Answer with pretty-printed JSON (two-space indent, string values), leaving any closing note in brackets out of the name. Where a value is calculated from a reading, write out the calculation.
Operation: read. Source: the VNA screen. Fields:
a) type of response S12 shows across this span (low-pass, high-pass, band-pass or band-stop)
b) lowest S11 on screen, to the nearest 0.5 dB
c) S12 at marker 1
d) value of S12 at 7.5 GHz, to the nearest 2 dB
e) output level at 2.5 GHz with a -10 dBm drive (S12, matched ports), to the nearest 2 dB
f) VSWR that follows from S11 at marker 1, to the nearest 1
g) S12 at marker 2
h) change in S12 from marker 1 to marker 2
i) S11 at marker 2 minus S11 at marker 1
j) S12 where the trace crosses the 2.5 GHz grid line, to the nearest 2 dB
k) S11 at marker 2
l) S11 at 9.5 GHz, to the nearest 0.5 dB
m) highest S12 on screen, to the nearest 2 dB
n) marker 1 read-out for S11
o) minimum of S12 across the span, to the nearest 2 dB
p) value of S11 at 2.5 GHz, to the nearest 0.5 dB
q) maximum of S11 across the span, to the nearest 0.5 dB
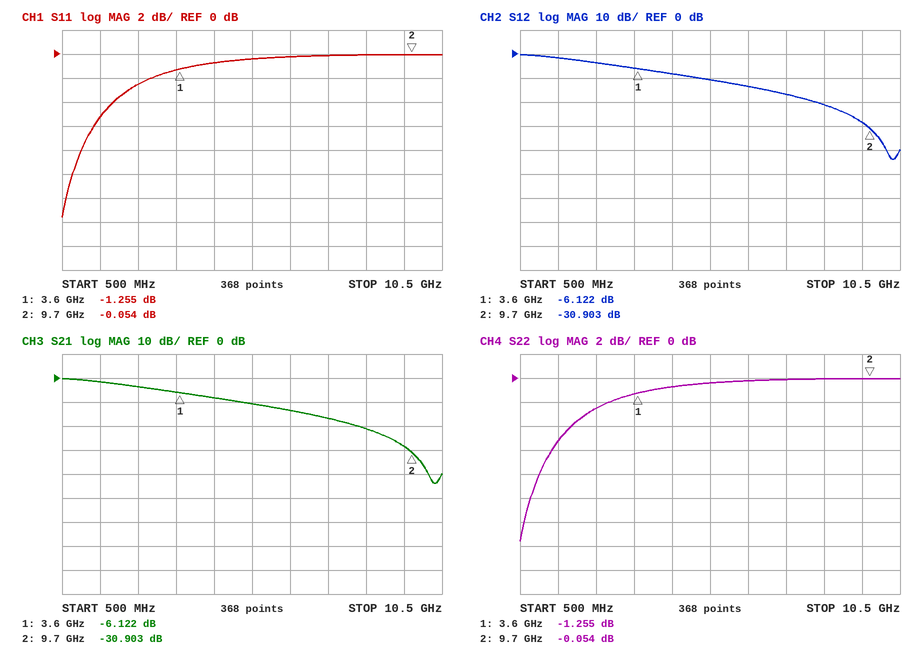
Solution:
{
  "type of response S12 shows across this span": "low-pass",
  "lowest S11 on screen, to the nearest 0.5 dB": "-13.5 dB",
  "S12 at marker 1": "-6.122 dB",
  "value of S12 at 7.5 GHz, to the nearest 2 dB": "-16 dB",
  "output level at 2.5 GHz with a -10 dBm drive (S12, matched ports), to the nearest 2 dB": "-10 dBm + (-4 dB) = -14 dBm",
  "VSWR that follows from S11 at marker 1, to the nearest 1": "(1 + 0.8655)/(1 − 0.8655) ≈ 14",
  "S12 at marker 2": "-30.903 dB",
  "change in S12 from marker 1 to marker 2": "-30.903 − (-6.122) = -24.781 dB",
  "S11 at marker 2 minus S11 at marker 1": "-0.054 − (-1.255) = 1.201 dB",
  "S12 where the trace crosses the 2.5 GHz grid line, to the nearest 2 dB": "-4 dB",
  "S11 at marker 2": "-0.054 dB",
  "S11 at 9.5 GHz, to the nearest 0.5 dB": "0.0 dB",
  "highest S12 on screen, to the nearest 2 dB": "0 dB",
  "marker 1 read-out for S11": "-1.255 dB",
  "minimum of S12 across the span, to the nearest 2 dB": "-44 dB",
  "value of S11 at 2.5 GHz, to the nearest 0.5 dB": "-2.5 dB",
  "maximum of S11 across the span, to the nearest 0.5 dB": "0.0 dB"
}
